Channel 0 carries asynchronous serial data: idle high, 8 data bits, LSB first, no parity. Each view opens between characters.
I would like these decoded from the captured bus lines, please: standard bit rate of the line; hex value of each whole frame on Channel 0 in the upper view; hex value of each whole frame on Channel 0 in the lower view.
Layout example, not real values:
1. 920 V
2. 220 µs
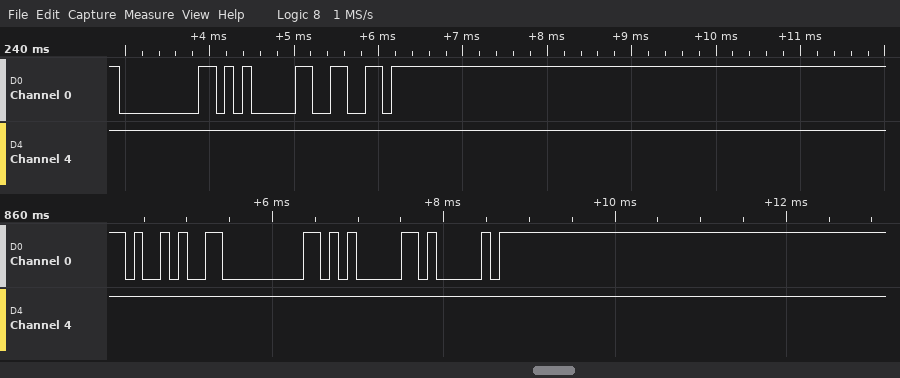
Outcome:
1. 9600 baud
2. 00, 05, 66
3. 29, 00, 05, 41
